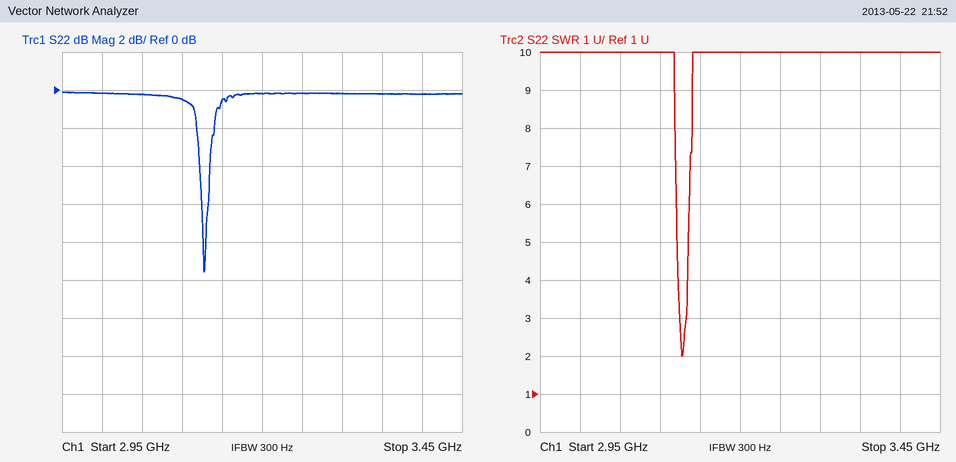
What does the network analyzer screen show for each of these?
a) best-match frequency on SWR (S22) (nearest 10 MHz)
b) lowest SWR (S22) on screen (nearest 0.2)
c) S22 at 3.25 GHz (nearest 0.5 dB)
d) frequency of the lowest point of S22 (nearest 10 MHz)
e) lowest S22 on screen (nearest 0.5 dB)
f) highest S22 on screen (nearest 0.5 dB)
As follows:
3.13 GHz
2.0
0.0 dB
3.13 GHz
-9.5 dB
0.0 dB
